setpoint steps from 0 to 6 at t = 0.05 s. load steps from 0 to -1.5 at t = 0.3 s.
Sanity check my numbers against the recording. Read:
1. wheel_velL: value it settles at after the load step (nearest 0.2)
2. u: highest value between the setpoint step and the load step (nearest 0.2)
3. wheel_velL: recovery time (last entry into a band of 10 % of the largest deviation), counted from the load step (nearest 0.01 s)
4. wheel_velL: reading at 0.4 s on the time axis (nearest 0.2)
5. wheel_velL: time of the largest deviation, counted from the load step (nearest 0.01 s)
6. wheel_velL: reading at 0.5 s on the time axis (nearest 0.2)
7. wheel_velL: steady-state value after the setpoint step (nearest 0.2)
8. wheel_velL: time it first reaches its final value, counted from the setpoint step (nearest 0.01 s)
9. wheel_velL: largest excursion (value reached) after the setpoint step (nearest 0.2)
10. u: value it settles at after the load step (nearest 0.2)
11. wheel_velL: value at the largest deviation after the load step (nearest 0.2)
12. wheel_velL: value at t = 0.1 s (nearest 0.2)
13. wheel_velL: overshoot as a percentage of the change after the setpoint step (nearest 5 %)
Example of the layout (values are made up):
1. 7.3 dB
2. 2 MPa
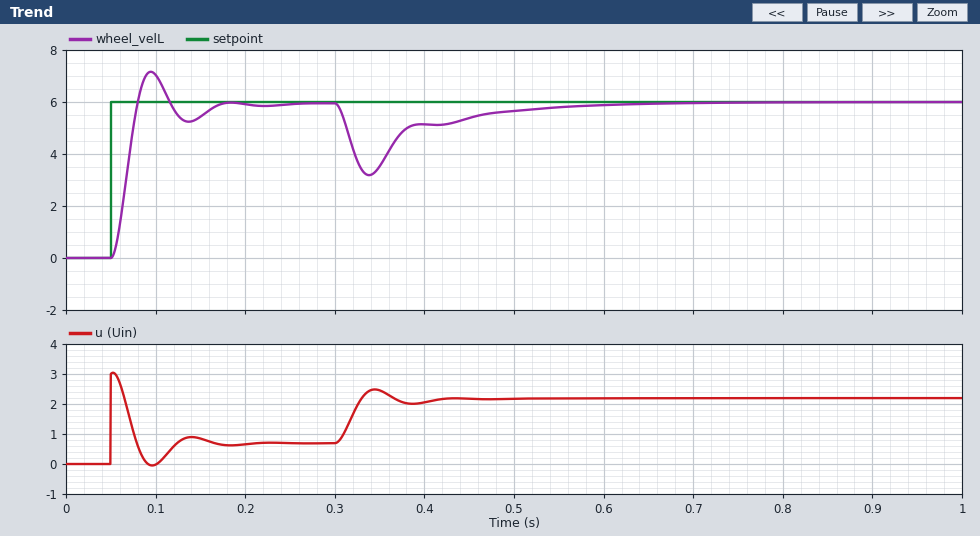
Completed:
1. 6.0
2. 3.0
3. 0.22 s
4. 5.2
5. 0.04 s
6. 5.6
7. 6.0
8. 0.03 s
9. 7.2
10. 2.2
11. 3.2
12. 7.0
13. 20 %
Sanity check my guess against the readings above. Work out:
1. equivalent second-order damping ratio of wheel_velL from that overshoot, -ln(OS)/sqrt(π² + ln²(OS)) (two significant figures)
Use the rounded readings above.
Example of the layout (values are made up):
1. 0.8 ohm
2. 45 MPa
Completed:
1. 0.46
